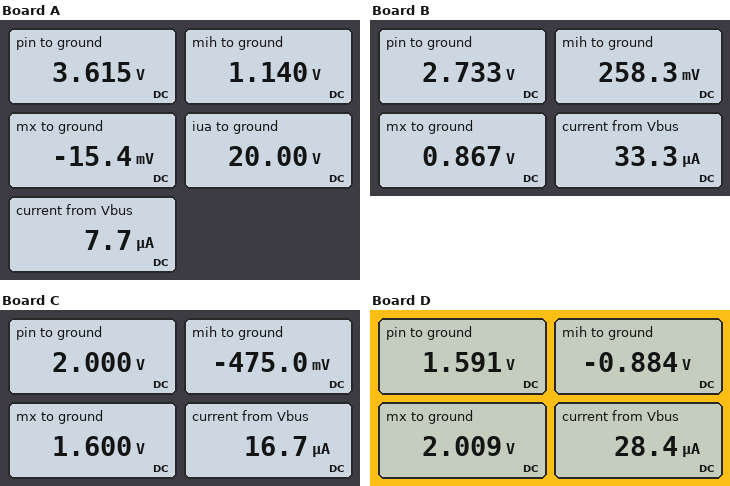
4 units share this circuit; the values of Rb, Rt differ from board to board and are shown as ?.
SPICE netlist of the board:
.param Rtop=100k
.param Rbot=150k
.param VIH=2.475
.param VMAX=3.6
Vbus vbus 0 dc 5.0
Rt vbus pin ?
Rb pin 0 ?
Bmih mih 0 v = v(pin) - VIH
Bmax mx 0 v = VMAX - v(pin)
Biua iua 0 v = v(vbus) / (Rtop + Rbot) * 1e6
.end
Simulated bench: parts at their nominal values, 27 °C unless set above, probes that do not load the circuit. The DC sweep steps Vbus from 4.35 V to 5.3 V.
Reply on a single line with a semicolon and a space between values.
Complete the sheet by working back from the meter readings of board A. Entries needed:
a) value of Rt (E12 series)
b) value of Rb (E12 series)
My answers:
180 kΩ; 470 kΩ
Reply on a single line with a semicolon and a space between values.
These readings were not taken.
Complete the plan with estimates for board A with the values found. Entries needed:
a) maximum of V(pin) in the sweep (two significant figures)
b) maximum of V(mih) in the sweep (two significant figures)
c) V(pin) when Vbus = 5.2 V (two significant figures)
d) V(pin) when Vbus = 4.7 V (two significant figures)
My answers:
3.8 V; 1.4 V; 3.8 V; 3.4 V
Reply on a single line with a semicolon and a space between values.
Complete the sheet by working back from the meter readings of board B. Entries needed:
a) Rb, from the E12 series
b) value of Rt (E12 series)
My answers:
82 kΩ; 68 kΩ
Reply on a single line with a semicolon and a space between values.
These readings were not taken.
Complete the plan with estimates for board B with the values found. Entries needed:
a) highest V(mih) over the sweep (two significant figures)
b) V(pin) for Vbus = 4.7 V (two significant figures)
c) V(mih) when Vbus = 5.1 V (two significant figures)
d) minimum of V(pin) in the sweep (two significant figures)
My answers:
420 mV; 2.6 V; 310 mV; 2.4 V
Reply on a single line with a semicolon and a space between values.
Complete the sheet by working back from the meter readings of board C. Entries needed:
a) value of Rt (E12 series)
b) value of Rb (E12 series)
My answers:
180 kΩ; 120 kΩ
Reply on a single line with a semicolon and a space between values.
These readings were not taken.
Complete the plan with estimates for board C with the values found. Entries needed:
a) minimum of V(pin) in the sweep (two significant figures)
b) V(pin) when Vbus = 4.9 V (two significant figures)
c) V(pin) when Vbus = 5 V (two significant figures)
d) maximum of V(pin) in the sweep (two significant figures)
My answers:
1.7 V; 2.0 V; 2.0 V; 2.1 V
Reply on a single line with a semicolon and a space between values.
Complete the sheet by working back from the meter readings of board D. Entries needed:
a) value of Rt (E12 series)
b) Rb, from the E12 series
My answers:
120 kΩ; 56 kΩ
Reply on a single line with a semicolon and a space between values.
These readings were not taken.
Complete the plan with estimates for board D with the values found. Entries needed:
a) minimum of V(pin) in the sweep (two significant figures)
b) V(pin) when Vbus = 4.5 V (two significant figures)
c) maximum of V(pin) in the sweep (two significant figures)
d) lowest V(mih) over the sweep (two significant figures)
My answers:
1.4 V; 1.4 V; 1.7 V; -1.1 V
